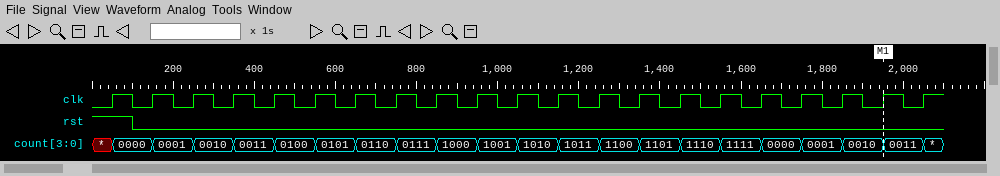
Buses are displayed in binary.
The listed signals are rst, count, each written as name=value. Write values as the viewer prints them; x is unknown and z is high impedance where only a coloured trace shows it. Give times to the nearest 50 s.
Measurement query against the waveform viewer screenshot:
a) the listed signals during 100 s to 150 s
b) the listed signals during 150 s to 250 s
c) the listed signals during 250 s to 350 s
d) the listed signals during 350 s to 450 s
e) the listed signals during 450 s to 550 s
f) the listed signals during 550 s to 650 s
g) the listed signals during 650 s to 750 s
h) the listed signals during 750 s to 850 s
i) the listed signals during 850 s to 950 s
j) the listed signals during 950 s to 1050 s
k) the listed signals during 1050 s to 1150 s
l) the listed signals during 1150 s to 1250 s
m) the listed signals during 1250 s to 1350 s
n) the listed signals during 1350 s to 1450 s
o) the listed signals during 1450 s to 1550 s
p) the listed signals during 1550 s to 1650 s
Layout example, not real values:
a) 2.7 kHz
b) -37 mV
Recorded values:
a) rst=0, count=0000
b) rst=0, count=0001
c) rst=0, count=0010
d) rst=0, count=0011
e) rst=0, count=0100
f) rst=0, count=0101
g) rst=0, count=0110
h) rst=0, count=0111
i) rst=0, count=1000
j) rst=0, count=1001
k) rst=0, count=1010
l) rst=0, count=1011
m) rst=0, count=1100
n) rst=0, count=1101
o) rst=0, count=1110
p) rst=0, count=1111
